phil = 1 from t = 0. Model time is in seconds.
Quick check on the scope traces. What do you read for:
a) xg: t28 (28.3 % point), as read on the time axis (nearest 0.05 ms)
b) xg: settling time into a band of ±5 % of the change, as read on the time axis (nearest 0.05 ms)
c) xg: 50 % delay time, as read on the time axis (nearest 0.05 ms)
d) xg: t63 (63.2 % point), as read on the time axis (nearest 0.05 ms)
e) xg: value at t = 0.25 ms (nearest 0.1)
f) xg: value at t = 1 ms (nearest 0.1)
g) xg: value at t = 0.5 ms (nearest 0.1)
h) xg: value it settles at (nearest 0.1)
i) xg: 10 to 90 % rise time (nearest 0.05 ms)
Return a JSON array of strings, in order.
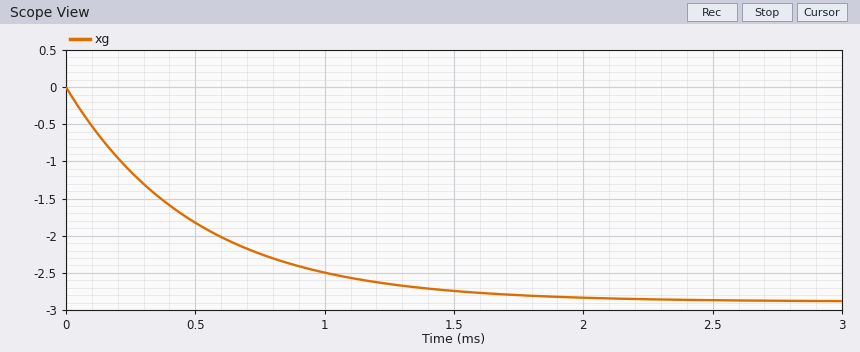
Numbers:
["0.15 ms", "1.50 ms", "0.35 ms", "0.50 ms", "-1.1", "-2.5", "-1.8", "-2.9", "1.10 ms"]
